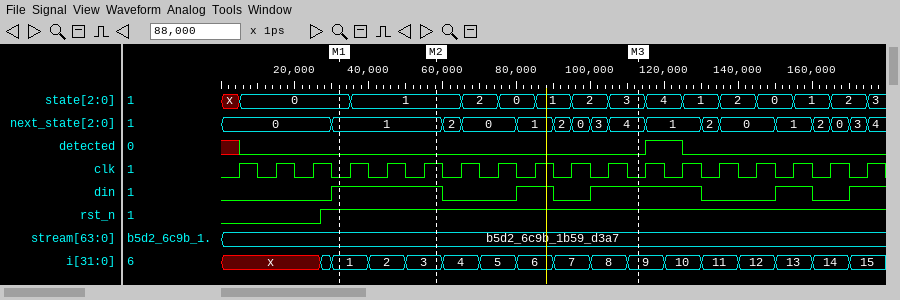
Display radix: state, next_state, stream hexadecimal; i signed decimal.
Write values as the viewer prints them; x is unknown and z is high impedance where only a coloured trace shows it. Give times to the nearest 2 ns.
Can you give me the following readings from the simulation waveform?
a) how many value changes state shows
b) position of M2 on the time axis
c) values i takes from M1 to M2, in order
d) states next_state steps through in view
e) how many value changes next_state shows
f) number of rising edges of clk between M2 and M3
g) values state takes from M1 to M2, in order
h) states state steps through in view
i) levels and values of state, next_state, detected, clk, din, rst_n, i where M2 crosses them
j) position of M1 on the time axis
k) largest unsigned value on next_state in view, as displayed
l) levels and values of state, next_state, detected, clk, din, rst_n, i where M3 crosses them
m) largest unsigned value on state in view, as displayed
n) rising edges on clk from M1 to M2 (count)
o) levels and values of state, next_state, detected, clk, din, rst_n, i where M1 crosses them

14
58 ns
1, 2, 3
0, 1, 2, 0, 1, 2, 0, 3, 4, 1, 2, 0, 1, 2, 0, 3, 4
16
5
0, 1
x, 0, 1, 2, 0, 1, 2, 3, 4, 1, 2, 0, 1, 2, 3
state=1, next_state=1, detected=0, clk=1, din=1, rst_n=1, i=3
32 ns
4
state=3, next_state=4, detected=0, clk=0, din=1, rst_n=1, i=9
4
3
state=0, next_state=1, detected=0, clk=0, din=1, rst_n=1, i=1
